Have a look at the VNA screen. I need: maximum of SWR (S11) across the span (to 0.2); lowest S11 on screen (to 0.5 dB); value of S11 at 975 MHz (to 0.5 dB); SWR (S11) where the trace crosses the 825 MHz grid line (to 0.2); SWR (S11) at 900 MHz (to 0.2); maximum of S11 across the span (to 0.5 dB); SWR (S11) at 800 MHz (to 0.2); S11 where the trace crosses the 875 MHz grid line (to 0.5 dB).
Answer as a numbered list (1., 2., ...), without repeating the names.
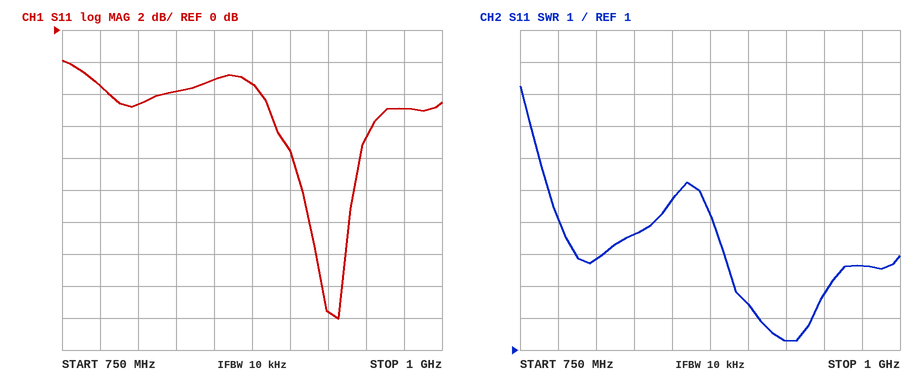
1. 9.2
2. -18.0 dB
3. -5.0 dB
4. 4.6
5. 2.4
6. -2.0 dB
7. 3.8
8. -3.5 dB
